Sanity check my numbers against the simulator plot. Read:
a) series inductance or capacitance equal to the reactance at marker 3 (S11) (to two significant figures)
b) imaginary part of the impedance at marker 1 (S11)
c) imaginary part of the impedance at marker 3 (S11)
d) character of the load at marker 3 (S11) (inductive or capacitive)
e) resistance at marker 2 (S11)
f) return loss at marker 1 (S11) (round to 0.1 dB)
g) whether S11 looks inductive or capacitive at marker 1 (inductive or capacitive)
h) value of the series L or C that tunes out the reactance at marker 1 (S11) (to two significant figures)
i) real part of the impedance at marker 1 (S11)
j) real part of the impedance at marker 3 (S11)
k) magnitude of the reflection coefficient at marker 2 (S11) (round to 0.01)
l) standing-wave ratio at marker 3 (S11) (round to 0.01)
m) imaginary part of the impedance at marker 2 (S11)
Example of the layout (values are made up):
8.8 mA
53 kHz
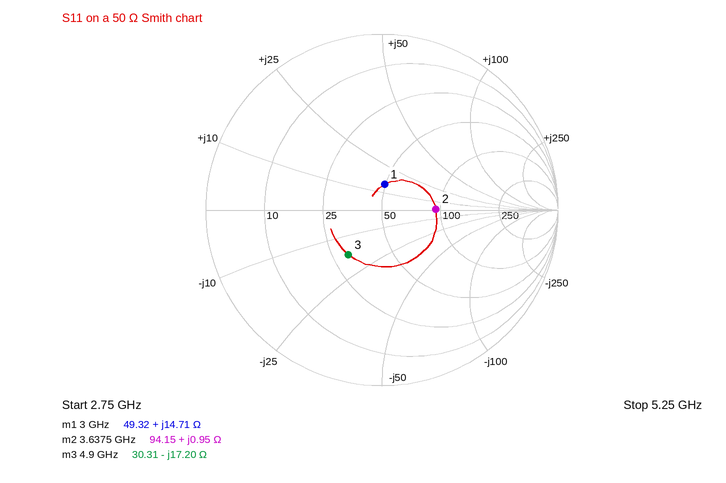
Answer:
1.9 pF
+14.71 Ω
-17.20 Ω
capacitive
94.15 Ω
16.7 dB
inductive
3.6 pF
49.32 Ω
30.31 Ω
0.31
1.93
+0.95 Ω
